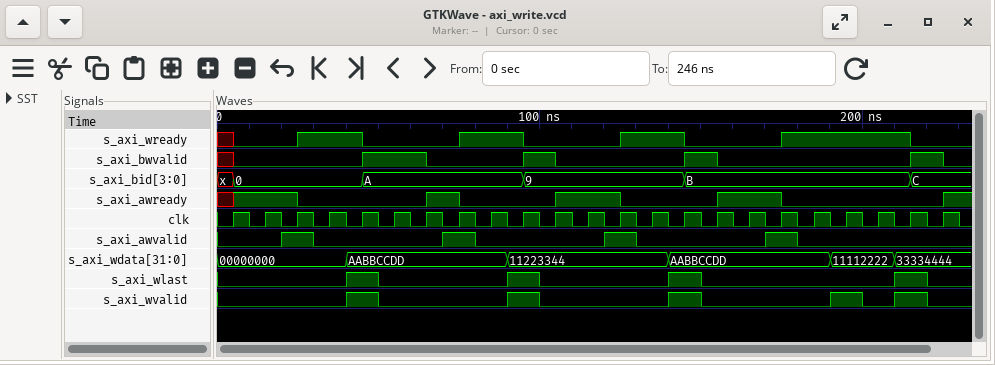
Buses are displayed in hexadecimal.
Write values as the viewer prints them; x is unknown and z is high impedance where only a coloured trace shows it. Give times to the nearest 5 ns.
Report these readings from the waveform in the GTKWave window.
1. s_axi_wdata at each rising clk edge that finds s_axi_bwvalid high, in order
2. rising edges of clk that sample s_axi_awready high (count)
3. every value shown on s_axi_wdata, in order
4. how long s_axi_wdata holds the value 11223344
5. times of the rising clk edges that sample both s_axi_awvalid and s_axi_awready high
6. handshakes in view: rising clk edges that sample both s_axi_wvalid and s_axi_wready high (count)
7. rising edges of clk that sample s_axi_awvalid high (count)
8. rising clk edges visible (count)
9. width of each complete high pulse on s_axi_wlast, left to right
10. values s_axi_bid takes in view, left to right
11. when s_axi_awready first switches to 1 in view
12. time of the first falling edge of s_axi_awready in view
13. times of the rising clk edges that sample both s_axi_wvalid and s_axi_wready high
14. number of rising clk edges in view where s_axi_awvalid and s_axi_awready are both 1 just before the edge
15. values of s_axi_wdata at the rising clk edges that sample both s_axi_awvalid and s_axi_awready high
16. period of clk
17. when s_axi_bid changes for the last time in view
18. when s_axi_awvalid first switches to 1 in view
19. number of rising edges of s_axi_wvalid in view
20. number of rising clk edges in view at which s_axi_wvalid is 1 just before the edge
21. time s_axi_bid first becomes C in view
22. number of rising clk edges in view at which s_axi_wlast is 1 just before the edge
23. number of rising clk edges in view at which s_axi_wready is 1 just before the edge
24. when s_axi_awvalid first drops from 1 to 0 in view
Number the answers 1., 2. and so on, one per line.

1. AABBCCDD, AABBCCDD, 11223344, AABBCCDD, 33334444
2. 7
3. 00000000, AABBCCDD, 11223344, AABBCCDD, 11112222, 33334444
4. 50 ns
5. 25 ns, 75 ns, 125 ns, 175 ns
6. 5
7. 4
8. 23
9. 10 ns, 10 ns, 10 ns, 10 ns
10. x, 0, A, 9, B, C
11. 5 ns
12. 25 ns
13. 45 ns, 95 ns, 145 ns, 195 ns, 215 ns
14. 4
15. 00000000, AABBCCDD, 11223344, AABBCCDD
16. 10 ns
17. 215 ns
18. 20 ns
19. 5
20. 5
21. 215 ns
22. 4
23. 10
24. 30 ns
